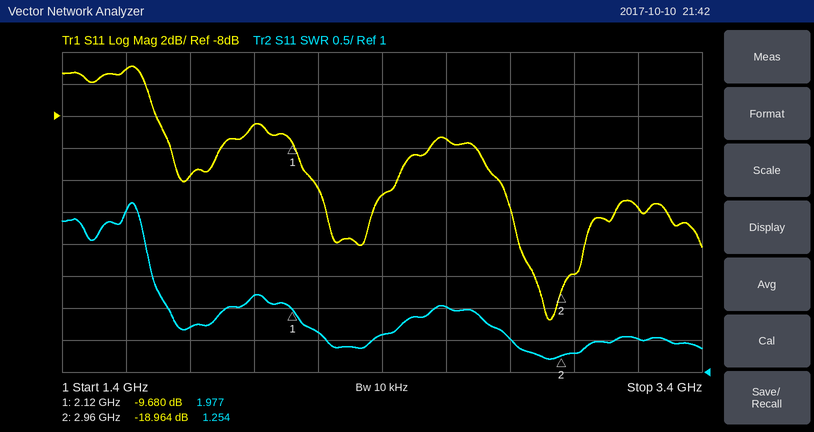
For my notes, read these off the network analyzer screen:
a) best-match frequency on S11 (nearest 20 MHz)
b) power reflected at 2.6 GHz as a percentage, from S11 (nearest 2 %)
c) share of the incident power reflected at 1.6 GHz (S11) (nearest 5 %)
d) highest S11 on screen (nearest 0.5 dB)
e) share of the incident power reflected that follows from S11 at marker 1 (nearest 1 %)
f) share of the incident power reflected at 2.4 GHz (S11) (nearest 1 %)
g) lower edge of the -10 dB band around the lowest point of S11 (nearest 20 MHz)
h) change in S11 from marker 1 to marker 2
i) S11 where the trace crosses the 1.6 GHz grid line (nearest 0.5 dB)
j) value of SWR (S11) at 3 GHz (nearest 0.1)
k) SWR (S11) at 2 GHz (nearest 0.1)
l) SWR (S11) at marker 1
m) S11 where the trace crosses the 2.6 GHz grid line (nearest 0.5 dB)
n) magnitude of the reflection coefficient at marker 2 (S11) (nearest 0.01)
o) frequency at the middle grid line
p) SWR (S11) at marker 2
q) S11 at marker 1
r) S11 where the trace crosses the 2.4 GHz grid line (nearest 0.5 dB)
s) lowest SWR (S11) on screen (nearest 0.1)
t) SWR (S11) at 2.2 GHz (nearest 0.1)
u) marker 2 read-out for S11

2.92 GHz
12 %
30 %
-5.0 dB
11 %
5 %
2.70 GHz
-9.284 dB
-5.0 dB
1.3
2.2
1.977
-9.5 dB
0.11
2.4 GHz
1.254
-9.680 dB
-13.0 dB
1.2
1.6
-18.964 dB
